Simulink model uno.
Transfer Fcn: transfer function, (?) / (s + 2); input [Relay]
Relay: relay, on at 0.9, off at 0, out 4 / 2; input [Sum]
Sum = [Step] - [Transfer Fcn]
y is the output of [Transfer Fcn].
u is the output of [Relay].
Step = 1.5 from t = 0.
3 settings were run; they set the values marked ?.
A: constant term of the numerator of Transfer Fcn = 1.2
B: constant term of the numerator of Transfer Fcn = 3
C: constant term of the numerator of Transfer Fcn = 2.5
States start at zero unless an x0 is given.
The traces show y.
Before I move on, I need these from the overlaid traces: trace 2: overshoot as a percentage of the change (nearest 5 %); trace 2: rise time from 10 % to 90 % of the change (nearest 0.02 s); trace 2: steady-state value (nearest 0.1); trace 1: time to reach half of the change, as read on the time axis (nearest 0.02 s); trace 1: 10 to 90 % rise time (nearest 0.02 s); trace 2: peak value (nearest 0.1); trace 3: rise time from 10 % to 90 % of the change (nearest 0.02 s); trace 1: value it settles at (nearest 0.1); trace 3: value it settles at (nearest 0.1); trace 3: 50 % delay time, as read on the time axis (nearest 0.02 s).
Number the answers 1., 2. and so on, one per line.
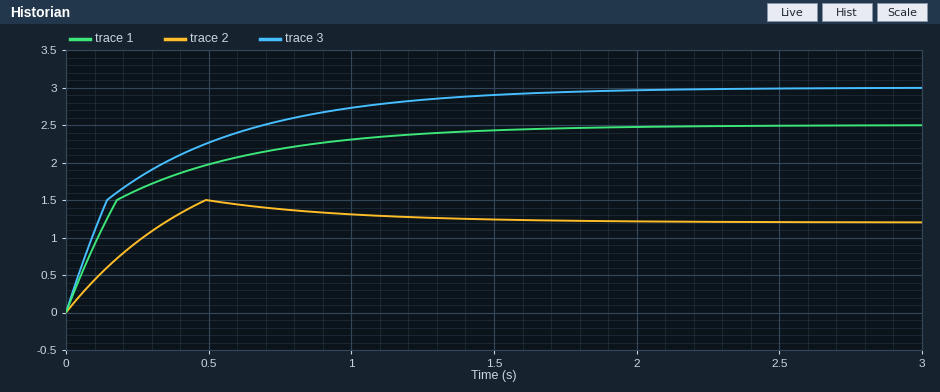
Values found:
1. 25 %
2. 0.28 s
3. 1.2
4. 0.14 s
5. 0.84 s
6. 1.5
7. 0.92 s
8. 2.5
9. 3.0
10. 0.14 s
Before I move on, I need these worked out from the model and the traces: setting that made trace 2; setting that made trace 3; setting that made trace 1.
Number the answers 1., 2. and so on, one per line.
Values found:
1. A
2. B
3. C
